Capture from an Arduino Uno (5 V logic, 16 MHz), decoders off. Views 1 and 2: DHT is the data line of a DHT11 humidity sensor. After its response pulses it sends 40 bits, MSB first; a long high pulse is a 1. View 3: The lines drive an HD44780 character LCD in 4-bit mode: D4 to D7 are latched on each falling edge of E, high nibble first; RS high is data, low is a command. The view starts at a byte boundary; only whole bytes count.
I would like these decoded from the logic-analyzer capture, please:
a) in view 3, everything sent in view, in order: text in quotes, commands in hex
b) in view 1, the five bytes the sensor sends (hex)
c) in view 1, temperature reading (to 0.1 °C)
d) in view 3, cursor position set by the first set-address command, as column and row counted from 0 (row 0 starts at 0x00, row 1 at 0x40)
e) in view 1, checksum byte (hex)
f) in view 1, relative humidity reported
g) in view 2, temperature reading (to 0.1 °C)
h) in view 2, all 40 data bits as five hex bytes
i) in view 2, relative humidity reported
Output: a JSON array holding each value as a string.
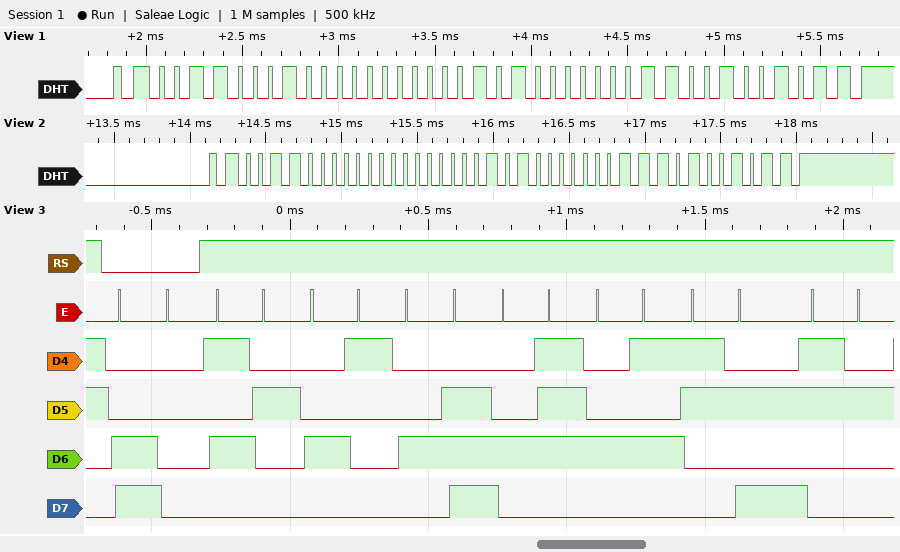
["0xC0 \"RANGE:2\"", "31 00 14 06 4B", "20.6 °C", "column 0, row 1", "0x4B", "49 %", "20.7 °C", "30 00 14 07 4B", "48 %"]
